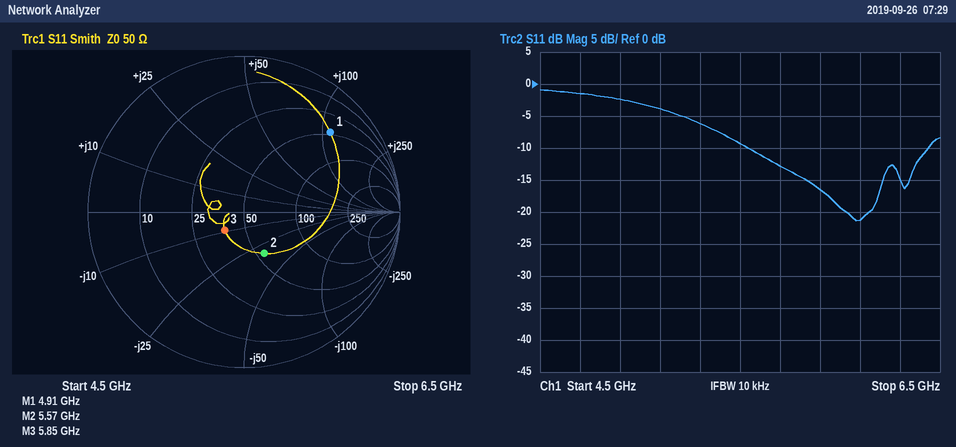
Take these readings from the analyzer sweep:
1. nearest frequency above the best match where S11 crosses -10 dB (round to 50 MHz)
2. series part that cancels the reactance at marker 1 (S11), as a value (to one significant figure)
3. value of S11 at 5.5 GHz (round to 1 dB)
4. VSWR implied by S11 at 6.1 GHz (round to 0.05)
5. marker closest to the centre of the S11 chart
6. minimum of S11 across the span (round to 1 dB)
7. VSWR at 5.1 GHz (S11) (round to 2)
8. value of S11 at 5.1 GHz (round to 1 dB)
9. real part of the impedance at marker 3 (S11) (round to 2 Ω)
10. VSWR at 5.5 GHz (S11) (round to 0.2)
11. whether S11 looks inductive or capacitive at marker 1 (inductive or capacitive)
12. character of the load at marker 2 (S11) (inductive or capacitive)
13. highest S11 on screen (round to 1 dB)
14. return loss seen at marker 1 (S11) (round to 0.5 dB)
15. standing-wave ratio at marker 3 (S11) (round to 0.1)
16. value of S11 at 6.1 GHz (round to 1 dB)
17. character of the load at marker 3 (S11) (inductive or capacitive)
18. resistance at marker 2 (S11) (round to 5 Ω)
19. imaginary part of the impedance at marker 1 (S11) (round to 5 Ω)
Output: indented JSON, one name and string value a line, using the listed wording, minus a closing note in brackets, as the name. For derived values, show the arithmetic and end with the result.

{
  "nearest frequency above the best match where S11 crosses -10 dB": "6.45 GHz",
  "series part that cancels the reactance at marker 1 (S11), as a value": "C = 1/(2π × 4.91 GHz × 110 Ω) ≈ 295 fF, so 300 fF to one significant figure",
  "value of S11 at 5.5 GHz": "-9 dB",
  "VSWR implied by S11 at 6.1 GHz": "|Γ| = 10^(-21/20) = 0.0891; VSWR = (1 + 0.0891)/(1 − 0.0891) ≈ 1.20",
  "marker closest to the centre of the S11 chart": "marker 3",
  "minimum of S11 across the span": "-21 dB",
  "VSWR at 5.1 GHz (S11)": "|Γ| = 10^(-4/20) = 0.6310; VSWR = (1 + 0.6310)/(1 − 0.6310) ≈ 4",
  "value of S11 at 5.1 GHz": "-4 dB",
  "real part of the impedance at marker 3 (S11)": "38 Ω",
  "VSWR at 5.5 GHz (S11)": "|Γ| = 10^(-9/20) = 0.3548; VSWR = (1 + 0.3548)/(1 − 0.3548) ≈ 2.10, so 2.0 to the nearest 0.2",
  "whether S11 looks inductive or capacitive at marker 1": "inductive",
  "character of the load at marker 2 (S11)": "capacitive",
  "highest S11 on screen": "-1 dB",
  "return loss seen at marker 1 (S11)": "2.5 dB",
  "standing-wave ratio at marker 3 (S11)": "1.4",
  "value of S11 at 6.1 GHz": "-21 dB",
  "character of the load at marker 3 (S11)": "capacitive",
  "resistance at marker 2 (S11)": "55 Ω",
  "imaginary part of the impedance at marker 1 (S11)": "+110 Ω"
}
